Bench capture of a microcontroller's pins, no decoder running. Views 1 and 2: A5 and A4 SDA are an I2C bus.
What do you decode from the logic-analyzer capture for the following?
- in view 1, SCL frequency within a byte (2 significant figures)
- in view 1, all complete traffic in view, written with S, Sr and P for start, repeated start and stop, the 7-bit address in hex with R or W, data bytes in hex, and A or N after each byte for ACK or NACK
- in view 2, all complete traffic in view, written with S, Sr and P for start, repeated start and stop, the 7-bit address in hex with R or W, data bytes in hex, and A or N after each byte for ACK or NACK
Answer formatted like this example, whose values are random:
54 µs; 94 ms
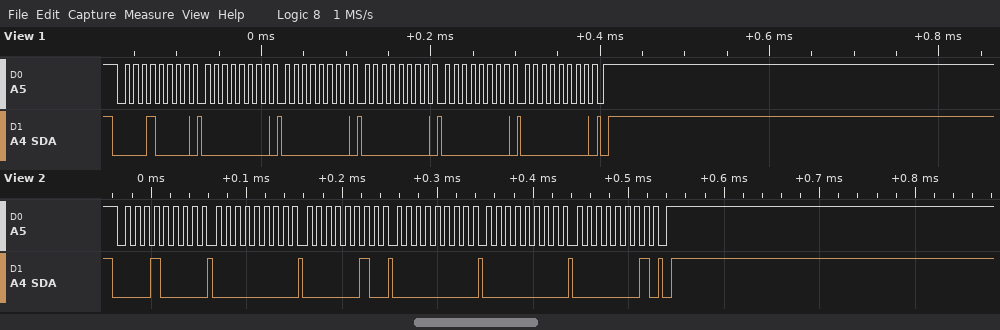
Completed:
100 kHz; S 08W A 00 A 00 A 00 A 00 A 00 A P; S 08W A 00 A 02 A 00 A 00 A 01 A P
